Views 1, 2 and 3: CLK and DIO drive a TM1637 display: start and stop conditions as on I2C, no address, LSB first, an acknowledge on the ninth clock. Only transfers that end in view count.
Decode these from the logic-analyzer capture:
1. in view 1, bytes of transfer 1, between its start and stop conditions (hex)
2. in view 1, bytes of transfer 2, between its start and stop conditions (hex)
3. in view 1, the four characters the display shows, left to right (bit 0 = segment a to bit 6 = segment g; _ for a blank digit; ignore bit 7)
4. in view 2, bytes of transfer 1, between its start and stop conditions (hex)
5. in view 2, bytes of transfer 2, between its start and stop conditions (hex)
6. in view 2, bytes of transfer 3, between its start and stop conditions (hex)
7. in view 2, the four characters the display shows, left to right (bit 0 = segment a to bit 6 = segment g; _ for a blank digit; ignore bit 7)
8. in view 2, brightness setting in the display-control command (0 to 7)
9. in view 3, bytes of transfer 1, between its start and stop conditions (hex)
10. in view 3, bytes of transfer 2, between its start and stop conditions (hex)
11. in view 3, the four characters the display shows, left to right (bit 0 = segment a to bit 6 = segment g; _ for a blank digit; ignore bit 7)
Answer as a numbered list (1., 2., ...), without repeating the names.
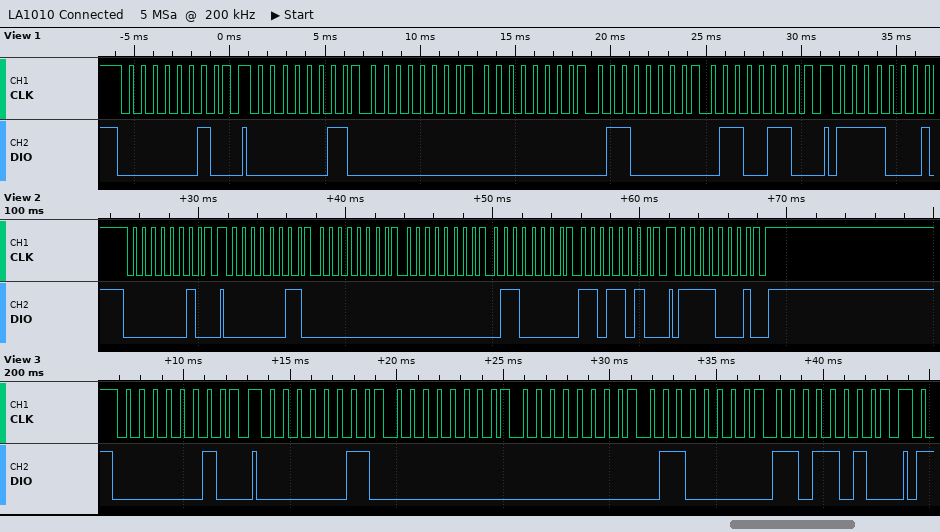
1. 40
2. C0 00 00 06 66
3. __14
4. 40
5. C0 00 00 06 5B
6. 8F
7. __12
8. 7
9. 40
10. C0 00 00 06 5B
11. __12
